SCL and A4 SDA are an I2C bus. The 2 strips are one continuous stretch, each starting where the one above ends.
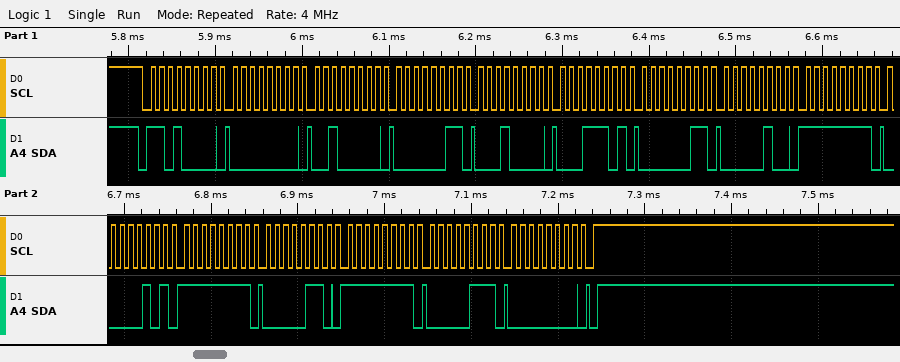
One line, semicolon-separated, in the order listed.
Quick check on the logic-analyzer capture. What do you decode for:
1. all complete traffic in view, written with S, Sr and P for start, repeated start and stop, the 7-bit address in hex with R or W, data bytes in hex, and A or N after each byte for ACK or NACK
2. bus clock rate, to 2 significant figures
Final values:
S 68W A 00 A 20 A 03 A 10 A 1D A 03 A 04 A FF A 05 A FF A 06 A FF A 07 A 00 A P; 100 kHz
